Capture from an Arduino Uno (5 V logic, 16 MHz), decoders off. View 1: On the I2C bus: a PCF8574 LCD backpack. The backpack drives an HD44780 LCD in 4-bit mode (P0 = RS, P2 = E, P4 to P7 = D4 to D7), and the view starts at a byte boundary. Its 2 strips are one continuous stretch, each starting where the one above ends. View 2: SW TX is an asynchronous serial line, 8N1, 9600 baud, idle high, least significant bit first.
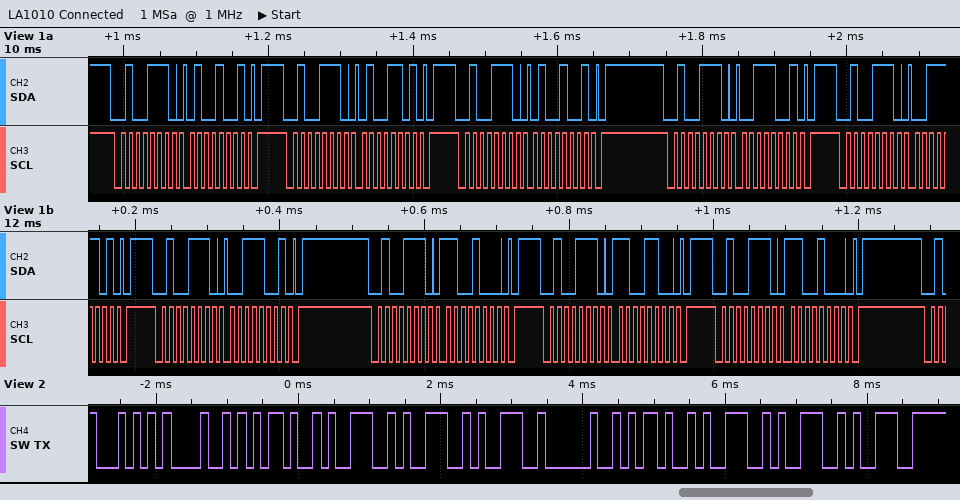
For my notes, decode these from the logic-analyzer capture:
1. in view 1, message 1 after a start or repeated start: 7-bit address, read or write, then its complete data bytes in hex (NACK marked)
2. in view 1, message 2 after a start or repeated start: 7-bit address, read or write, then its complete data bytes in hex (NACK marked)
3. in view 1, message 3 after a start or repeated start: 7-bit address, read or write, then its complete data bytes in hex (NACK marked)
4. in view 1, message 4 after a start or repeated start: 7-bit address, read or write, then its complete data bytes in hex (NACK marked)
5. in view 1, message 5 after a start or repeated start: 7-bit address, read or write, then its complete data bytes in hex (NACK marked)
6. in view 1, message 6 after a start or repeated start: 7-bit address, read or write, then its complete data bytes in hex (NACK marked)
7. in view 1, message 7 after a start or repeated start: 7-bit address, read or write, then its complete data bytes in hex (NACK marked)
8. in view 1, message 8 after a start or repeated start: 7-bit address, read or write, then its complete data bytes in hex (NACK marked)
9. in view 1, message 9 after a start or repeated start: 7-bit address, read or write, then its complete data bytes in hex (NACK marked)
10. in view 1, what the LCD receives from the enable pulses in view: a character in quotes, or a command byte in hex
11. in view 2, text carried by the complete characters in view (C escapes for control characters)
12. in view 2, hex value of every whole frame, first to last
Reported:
0x27 write: 49
0x27 write: 4D
0x27 write: 49
0x27 write: 39
0x27 write: 3D
0x27 write: 39
0x27 write: C8
0x27 write: CC
0x27 write: C8
'C'
"TH-999 -999"
0x54 0x48 0x2D 0x39 0x39 0x39 0x20 0x2D 0x39 0x39 0x39
